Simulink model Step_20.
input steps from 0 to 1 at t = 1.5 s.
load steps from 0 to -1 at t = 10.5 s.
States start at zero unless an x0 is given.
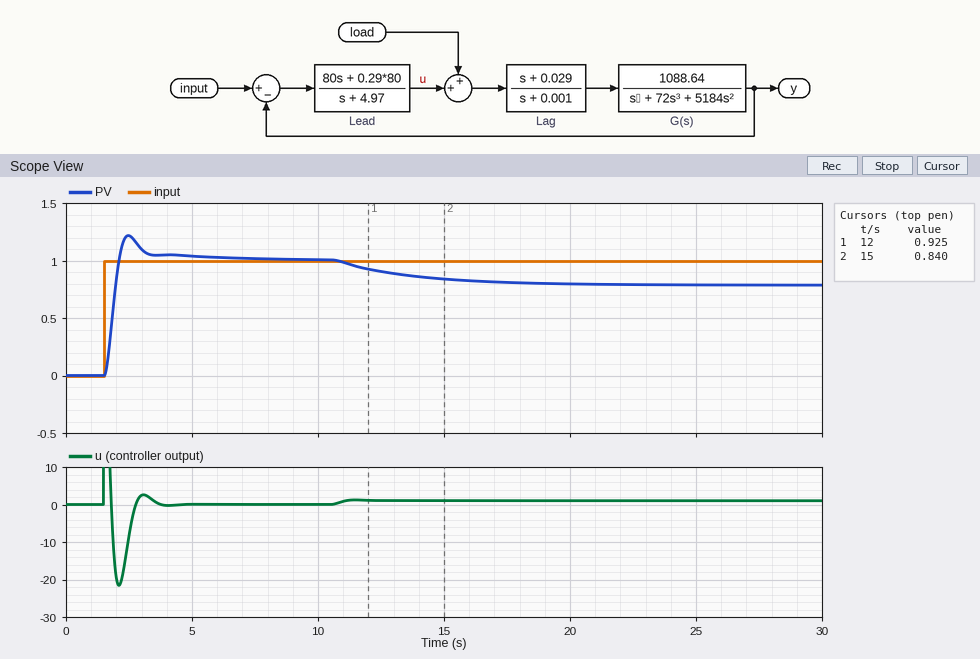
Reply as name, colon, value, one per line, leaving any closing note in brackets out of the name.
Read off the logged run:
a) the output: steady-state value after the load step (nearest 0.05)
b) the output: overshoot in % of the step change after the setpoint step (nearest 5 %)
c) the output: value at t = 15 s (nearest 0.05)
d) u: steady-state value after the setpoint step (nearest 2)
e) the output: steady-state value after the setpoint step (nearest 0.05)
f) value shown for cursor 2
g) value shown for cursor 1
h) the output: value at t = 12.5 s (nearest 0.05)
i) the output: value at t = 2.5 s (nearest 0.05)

the output: steady-state value after the load step: 0.80
the output: overshoot in % of the step change after the setpoint step: 20 %
the output: value at t = 15 s: 0.85
u: steady-state value after the setpoint step: 0
the output: steady-state value after the setpoint step: 1.00
value shown for cursor 2: 0.840
value shown for cursor 1: 0.925
the output: value at t = 12.5 s: 0.90
the output: value at t = 2.5 s: 1.20
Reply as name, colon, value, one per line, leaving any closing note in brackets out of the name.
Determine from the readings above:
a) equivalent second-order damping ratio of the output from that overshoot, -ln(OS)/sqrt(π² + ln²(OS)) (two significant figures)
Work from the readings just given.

equivalent second-order damping ratio of the output from that overshoot, -ln(OS)/sqrt(π² + ln²(OS)): 0.46
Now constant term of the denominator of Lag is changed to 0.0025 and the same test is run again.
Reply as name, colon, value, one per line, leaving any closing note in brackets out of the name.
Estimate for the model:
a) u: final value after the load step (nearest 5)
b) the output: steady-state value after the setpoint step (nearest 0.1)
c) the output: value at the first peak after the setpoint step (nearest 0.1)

u: final value after the load step: 0
the output: steady-state value after the setpoint step: 1.0
the output: value at the first peak after the setpoint step: 1.2
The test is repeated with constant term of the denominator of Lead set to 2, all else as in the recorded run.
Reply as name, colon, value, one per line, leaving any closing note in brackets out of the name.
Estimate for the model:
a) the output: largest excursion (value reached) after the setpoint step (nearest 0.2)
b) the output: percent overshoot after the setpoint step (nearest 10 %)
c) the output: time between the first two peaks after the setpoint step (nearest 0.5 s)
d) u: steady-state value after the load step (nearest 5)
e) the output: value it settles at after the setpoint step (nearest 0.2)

the output: largest excursion (value reached) after the setpoint step: 1.6
the output: percent overshoot after the setpoint step: 60 %
the output: time between the first two peaks after the setpoint step: 1.5 s
u: steady-state value after the load step: 0
the output: value it settles at after the setpoint step: 1.0
